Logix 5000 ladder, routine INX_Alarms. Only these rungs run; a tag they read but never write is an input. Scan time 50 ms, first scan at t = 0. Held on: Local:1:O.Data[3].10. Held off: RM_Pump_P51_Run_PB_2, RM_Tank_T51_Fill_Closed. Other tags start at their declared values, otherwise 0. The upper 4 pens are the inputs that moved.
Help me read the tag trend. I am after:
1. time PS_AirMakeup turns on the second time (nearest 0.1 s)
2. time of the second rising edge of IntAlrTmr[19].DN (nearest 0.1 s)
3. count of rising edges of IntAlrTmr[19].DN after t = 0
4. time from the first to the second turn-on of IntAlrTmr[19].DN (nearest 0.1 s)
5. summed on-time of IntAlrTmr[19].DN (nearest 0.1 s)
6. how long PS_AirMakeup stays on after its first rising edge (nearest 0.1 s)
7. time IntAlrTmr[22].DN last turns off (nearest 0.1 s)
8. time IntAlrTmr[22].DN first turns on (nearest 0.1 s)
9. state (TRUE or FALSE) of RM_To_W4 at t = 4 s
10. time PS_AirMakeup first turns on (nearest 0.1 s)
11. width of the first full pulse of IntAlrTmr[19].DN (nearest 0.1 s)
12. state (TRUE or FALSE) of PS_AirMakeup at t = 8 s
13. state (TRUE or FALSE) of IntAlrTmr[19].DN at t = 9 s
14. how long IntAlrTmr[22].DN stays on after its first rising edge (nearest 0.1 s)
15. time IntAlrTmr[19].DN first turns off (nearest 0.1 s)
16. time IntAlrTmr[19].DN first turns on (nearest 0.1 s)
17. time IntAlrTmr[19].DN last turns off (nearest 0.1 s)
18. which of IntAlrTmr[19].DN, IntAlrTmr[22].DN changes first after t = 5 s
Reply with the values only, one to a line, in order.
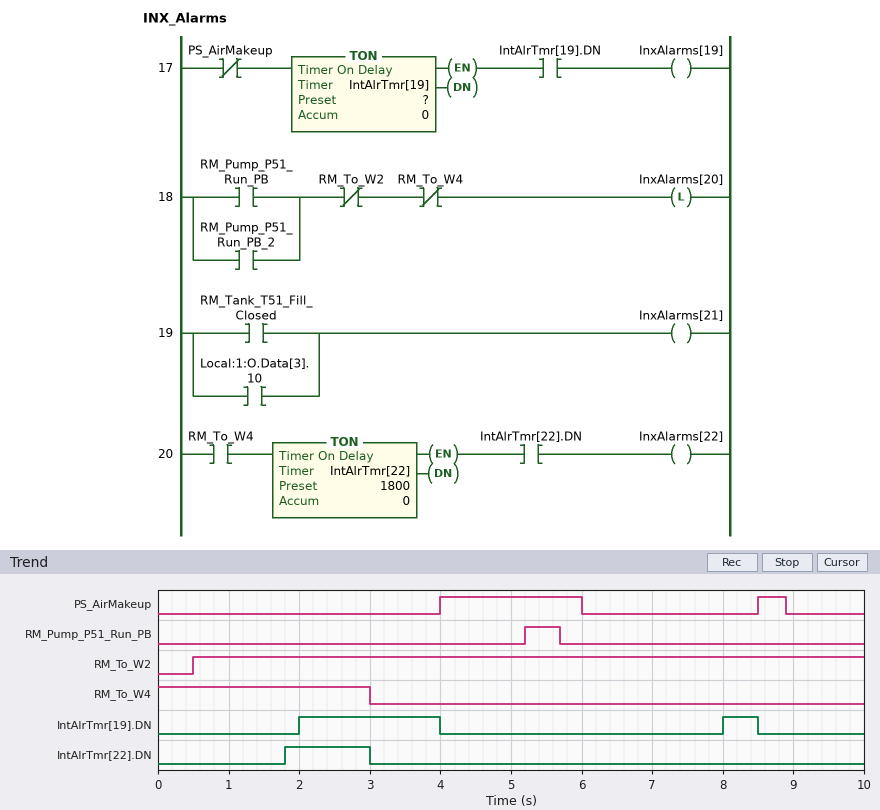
8.5 s
8.0 s
2
6.0 s
2.5 s
2.0 s
3.0 s
1.8 s
FALSE
4.0 s
2.0 s
FALSE
FALSE
1.2 s
4.0 s
2.0 s
8.5 s
IntAlrTmr[19].DN
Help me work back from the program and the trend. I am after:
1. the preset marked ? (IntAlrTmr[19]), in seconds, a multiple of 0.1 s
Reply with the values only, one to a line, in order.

2.0 s
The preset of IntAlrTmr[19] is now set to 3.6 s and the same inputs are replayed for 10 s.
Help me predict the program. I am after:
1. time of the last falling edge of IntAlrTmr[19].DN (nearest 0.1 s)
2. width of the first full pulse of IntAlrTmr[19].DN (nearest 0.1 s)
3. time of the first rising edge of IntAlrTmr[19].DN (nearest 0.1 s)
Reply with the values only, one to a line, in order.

4.0 s
0.4 s
3.6 s
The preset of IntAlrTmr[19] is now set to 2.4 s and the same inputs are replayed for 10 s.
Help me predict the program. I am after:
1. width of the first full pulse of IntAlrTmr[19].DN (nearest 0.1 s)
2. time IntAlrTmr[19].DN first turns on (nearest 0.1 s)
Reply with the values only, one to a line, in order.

1.6 s
2.4 s
